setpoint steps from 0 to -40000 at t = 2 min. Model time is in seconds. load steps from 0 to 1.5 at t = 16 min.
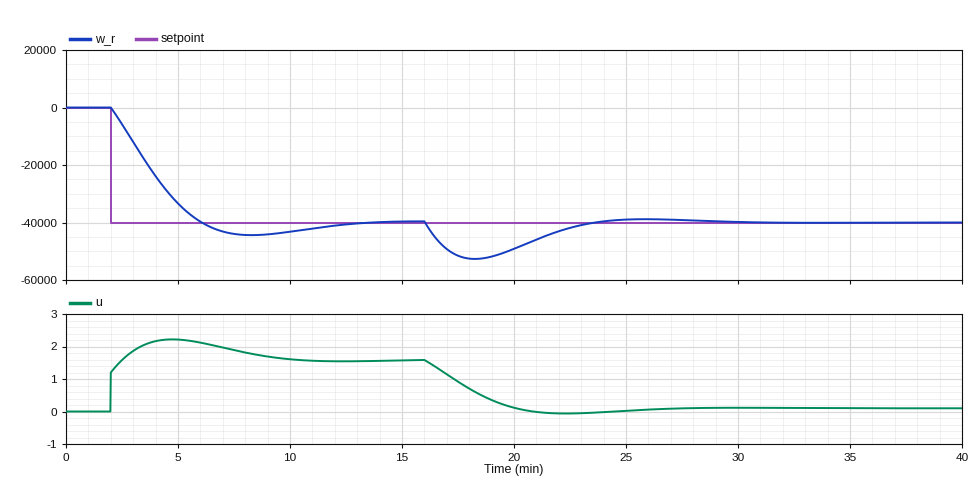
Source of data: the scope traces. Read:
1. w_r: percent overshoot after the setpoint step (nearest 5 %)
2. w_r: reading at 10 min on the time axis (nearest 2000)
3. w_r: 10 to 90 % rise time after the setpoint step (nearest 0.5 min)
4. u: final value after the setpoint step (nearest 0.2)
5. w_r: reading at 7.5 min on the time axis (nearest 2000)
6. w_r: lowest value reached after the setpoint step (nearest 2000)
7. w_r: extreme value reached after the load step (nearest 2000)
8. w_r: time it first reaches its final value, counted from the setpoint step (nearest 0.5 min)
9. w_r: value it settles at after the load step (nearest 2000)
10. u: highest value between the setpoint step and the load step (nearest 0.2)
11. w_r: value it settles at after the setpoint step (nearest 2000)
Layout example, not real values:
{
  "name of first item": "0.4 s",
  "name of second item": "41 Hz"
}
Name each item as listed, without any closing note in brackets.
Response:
{
  "w_r: percent overshoot after the setpoint step": "10 %",
  "w_r: reading at 10 min on the time axis": "-44000",
  "w_r: 10 to 90 % rise time after the setpoint step": "3.0 min",
  "u: final value after the setpoint step": "1.6",
  "w_r: reading at 7.5 min on the time axis": "-44000",
  "w_r: lowest value reached after the setpoint step": "-44000",
  "w_r: extreme value reached after the load step": "-52000",
  "w_r: time it first reaches its final value, counted from the setpoint step": "4.0 min",
  "w_r: value it settles at after the load step": "-40000",
  "u: highest value between the setpoint step and the load step": "2.2",
  "w_r: value it settles at after the setpoint step": "-40000"
}
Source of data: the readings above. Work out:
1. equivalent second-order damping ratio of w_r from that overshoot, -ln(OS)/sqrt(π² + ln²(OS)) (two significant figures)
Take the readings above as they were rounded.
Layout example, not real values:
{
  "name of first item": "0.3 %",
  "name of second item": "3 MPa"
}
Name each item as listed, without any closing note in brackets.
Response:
{
  "equivalent second-order damping ratio of w_r from that overshoot, -ln(OS)/sqrt(π² + ln²(OS))": "0.59"
}
